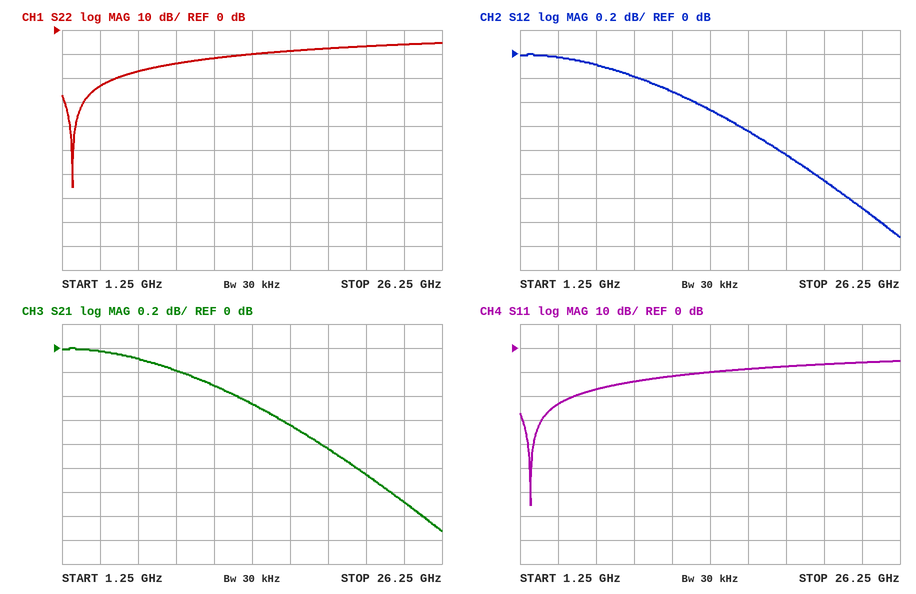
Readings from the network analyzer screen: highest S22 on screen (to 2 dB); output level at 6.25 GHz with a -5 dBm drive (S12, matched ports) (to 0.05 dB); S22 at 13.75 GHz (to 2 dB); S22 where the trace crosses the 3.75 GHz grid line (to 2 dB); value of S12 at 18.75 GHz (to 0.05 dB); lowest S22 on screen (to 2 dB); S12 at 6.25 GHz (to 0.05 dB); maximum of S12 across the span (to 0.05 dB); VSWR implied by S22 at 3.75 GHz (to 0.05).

-6 dB
-5.10 dBm
-10 dB
-24 dB
-0.85 dB
-66 dB
-0.10 dB
0.00 dB
1.15
